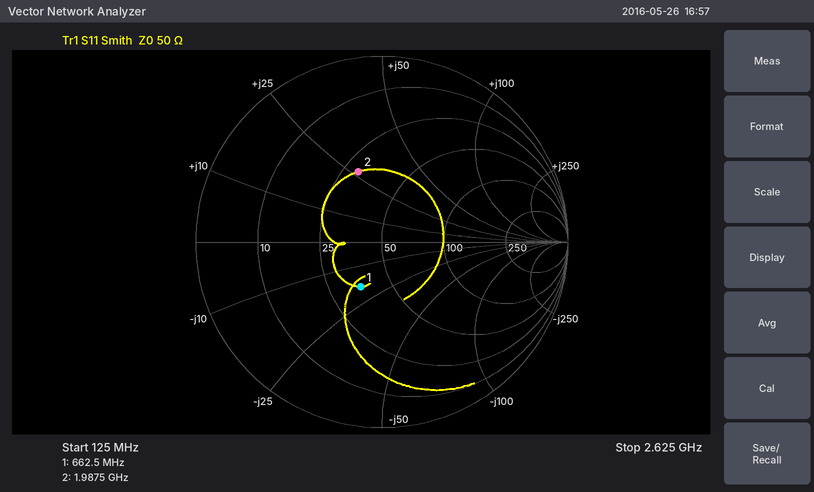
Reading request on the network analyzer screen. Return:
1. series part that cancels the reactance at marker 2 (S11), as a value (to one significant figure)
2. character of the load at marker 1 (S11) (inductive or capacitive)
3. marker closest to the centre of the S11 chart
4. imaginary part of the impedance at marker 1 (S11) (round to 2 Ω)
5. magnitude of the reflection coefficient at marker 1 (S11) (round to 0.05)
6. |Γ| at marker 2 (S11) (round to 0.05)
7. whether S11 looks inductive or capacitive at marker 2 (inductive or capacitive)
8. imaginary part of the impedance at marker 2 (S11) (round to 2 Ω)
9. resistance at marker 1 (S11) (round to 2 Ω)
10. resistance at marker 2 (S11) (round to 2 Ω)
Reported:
3 pF
capacitive
marker 1
-18 Ω
0.25
0.40
inductive
+26 Ω
36 Ω
30 Ω
